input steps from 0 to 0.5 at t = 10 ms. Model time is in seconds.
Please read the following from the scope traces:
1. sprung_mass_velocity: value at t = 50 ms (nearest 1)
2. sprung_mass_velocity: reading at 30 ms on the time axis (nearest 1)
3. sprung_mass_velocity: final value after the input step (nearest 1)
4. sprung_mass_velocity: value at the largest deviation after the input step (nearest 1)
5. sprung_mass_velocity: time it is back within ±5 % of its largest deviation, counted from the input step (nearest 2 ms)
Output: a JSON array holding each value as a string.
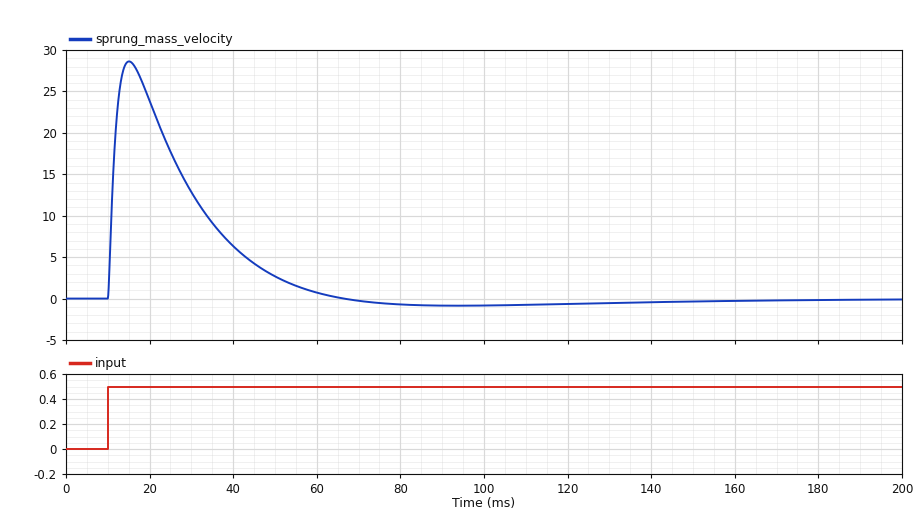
["3", "13", "0", "29", "46 ms"]
